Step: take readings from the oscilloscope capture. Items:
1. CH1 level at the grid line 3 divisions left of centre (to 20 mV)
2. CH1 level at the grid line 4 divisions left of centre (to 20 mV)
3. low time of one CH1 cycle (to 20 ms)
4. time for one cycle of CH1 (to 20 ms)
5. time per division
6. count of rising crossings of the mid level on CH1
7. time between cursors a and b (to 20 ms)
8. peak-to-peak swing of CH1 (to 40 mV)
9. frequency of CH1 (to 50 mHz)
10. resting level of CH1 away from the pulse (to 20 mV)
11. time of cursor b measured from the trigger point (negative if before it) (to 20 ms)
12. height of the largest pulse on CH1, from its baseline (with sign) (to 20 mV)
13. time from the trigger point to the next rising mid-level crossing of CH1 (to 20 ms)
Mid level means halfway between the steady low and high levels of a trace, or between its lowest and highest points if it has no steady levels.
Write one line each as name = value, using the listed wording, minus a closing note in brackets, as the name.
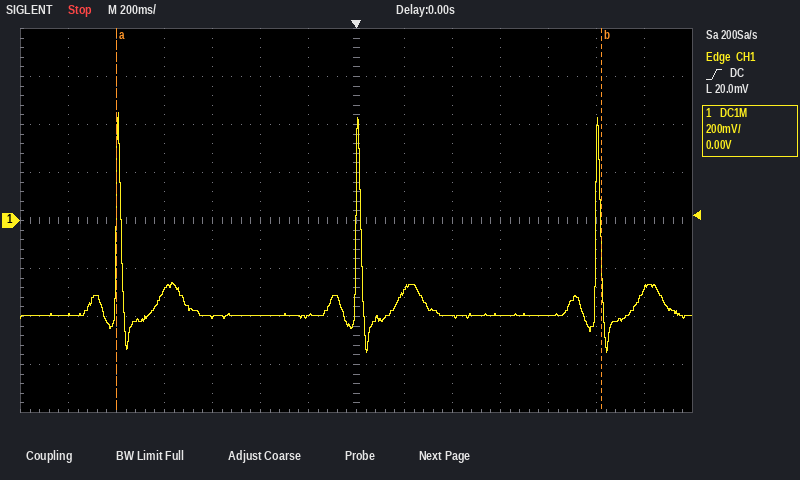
CH1 level at the grid line 3 divisions left of centre = -400 mV
CH1 level at the grid line 4 divisions left of centre = -300 mV
low time of one CH1 cycle = 980 ms
time for one cycle of CH1 = 1.00 s
time per division = 200 ms
count of rising crossings of the mid level on CH1 = 3
time between cursors a and b = 2.02 s
peak-to-peak swing of CH1 = 1.00 V
frequency of CH1 = 1.00 Hz
resting level of CH1 away from the pulse = -400 mV
time of cursor b measured from the trigger point (negative if before it) = +1.02 s
height of the largest pulse on CH1, from its baseline (with sign) = +840 mV
time from the trigger point to the next rising mid-level crossing of CH1 = 1.00 s
